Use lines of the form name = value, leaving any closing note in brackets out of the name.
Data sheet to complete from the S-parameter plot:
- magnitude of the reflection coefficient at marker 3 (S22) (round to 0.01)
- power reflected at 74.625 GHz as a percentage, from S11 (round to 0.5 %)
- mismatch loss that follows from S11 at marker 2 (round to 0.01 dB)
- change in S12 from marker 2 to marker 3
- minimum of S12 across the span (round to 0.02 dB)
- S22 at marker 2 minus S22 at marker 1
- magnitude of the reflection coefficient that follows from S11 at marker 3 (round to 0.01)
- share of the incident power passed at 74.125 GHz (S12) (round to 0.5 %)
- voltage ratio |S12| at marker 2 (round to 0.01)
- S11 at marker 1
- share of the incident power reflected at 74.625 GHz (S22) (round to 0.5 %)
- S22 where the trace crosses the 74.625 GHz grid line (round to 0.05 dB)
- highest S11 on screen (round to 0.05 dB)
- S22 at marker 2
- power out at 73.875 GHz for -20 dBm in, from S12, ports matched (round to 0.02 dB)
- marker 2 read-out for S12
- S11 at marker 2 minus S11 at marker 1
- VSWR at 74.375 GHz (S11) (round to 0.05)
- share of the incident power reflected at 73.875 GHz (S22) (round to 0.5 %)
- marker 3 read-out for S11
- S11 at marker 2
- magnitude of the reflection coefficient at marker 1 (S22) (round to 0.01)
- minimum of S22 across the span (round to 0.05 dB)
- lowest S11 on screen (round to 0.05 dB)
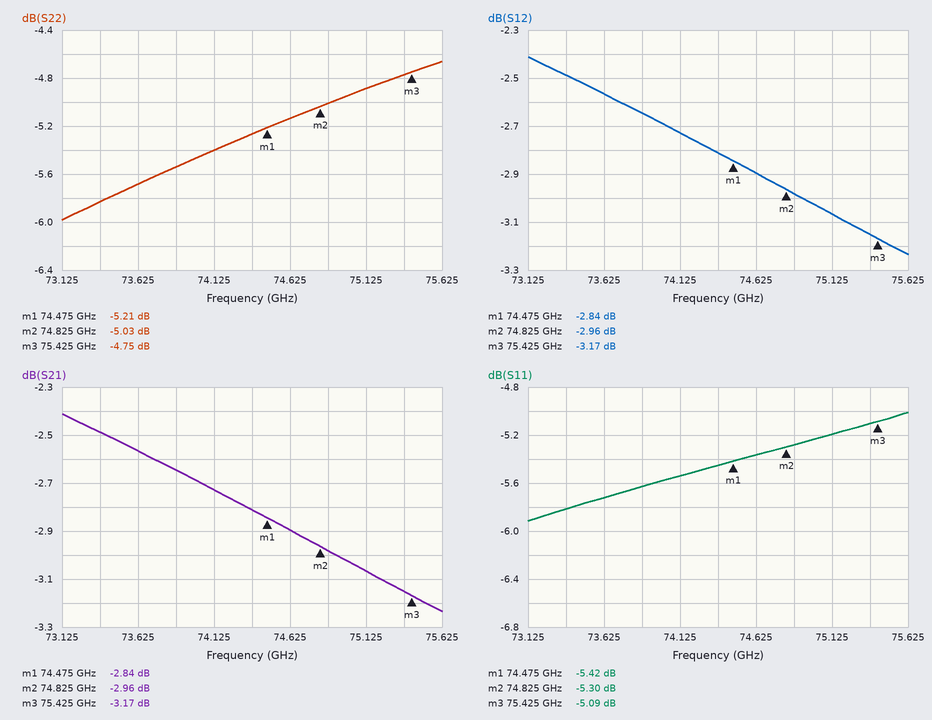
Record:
magnitude of the reflection coefficient at marker 3 (S22) = 0.58
power reflected at 74.625 GHz as a percentage, from S11 = 29.0 %
mismatch loss that follows from S11 at marker 2 = 1.52 dB
change in S12 from marker 2 to marker 3 = -0.21 dB
minimum of S12 across the span = -3.24 dB
S22 at marker 2 minus S22 at marker 1 = 0.18 dB
magnitude of the reflection coefficient that follows from S11 at marker 3 = 0.56
share of the incident power passed at 74.125 GHz (S12) = 53.5 %
voltage ratio |S12| at marker 2 = 0.71
S11 at marker 1 = -5.42 dB
share of the incident power reflected at 74.625 GHz (S22) = 30.5 %
S22 where the trace crosses the 74.625 GHz grid line = -5.15 dB
highest S11 on screen = -5.00 dB
S22 at marker 2 = -5.03 dB
power out at 73.875 GHz for -20 dBm in, from S12, ports matched = -22.64 dBm
marker 2 read-out for S12 = -2.96 dB
S11 at marker 2 minus S11 at marker 1 = 0.12 dB
VSWR at 74.375 GHz (S11) = 3.30
share of the incident power reflected at 73.875 GHz (S22) = 28.0 %
marker 3 read-out for S11 = -5.09 dB
S11 at marker 2 = -5.30 dB
magnitude of the reflection coefficient at marker 1 (S22) = 0.55
minimum of S22 across the span = -6.00 dB
lowest S11 on screen = -5.90 dB
